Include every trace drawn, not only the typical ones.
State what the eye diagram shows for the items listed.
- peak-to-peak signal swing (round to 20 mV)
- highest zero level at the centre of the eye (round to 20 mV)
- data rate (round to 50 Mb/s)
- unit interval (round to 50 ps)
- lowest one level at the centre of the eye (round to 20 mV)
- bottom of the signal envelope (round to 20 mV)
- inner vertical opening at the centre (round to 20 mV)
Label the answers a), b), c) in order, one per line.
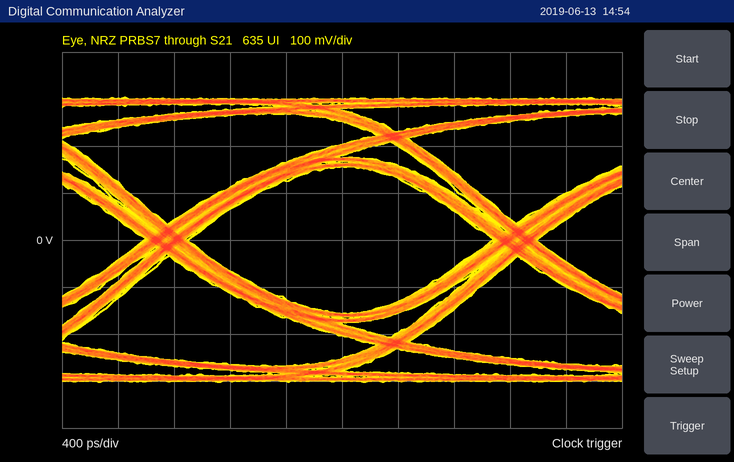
a) 600 mV
b) -160 mV
c) 400 Mb/s
d) 2.50 ns
e) 160 mV
f) -300 mV
g) 320 mV
